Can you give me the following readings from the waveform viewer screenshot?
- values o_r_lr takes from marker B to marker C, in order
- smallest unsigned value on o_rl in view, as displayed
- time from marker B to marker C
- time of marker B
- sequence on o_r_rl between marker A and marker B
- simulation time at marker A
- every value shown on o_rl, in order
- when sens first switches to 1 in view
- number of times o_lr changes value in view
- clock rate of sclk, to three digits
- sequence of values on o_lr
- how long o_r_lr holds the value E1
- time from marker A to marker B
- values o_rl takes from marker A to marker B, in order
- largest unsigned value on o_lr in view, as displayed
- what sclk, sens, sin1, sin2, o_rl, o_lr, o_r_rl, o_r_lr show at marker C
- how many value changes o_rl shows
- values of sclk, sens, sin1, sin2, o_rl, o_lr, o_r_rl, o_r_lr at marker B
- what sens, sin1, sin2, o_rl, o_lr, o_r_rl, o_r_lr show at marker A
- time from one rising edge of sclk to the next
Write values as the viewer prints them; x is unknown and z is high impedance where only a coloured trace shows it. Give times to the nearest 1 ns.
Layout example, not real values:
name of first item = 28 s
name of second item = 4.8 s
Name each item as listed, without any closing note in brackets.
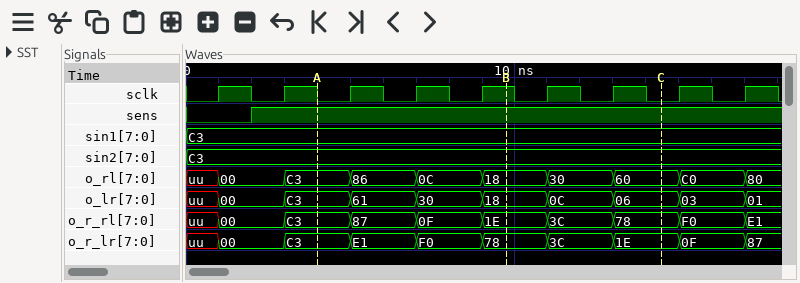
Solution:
values o_r_lr takes from marker B to marker C, in order = 78, 3C, 1E
smallest unsigned value on o_rl in view, as displayed = 00
time from marker B to marker C = 5 ns
time of marker B = 10 ns
sequence on o_r_rl between marker A and marker B = C3, 87, 0F, 1E
simulation time at marker A = 4 ns
every value shown on o_rl, in order = uu, 00, C3, 86, 0C, 18, 30, 60, C0, 80
when sens first switches to 1 in view = 2 ns
number of times o_lr changes value in view = 9
clock rate of sclk, to three digits = 500 MHz
sequence of values on o_lr = uu, 00, C3, 61, 30, 18, 0C, 06, 03, 01
how long o_r_lr holds the value E1 = 2 ns
time from marker A to marker B = 6 ns
values o_rl takes from marker A to marker B, in order = C3, 86, 0C, 18
largest unsigned value on o_lr in view, as displayed = C3
what sclk, sens, sin1, sin2, o_rl, o_lr, o_r_rl, o_r_lr show at marker C = sclk=0, sens=1, sin1=C3, sin2=C3, o_rl=60, o_lr=06, o_r_rl=78, o_r_lr=1E
how many value changes o_rl shows = 9
values of sclk, sens, sin1, sin2, o_rl, o_lr, o_r_rl, o_r_lr at marker B = sclk=1, sens=1, sin1=C3, sin2=C3, o_rl=18, o_lr=18, o_r_rl=1E, o_r_lr=78
what sens, sin1, sin2, o_rl, o_lr, o_r_rl, o_r_lr show at marker A = sens=1, sin1=C3, sin2=C3, o_rl=C3, o_lr=C3, o_r_rl=C3, o_r_lr=C3
time from one rising edge of sclk to the next = 2 ns
